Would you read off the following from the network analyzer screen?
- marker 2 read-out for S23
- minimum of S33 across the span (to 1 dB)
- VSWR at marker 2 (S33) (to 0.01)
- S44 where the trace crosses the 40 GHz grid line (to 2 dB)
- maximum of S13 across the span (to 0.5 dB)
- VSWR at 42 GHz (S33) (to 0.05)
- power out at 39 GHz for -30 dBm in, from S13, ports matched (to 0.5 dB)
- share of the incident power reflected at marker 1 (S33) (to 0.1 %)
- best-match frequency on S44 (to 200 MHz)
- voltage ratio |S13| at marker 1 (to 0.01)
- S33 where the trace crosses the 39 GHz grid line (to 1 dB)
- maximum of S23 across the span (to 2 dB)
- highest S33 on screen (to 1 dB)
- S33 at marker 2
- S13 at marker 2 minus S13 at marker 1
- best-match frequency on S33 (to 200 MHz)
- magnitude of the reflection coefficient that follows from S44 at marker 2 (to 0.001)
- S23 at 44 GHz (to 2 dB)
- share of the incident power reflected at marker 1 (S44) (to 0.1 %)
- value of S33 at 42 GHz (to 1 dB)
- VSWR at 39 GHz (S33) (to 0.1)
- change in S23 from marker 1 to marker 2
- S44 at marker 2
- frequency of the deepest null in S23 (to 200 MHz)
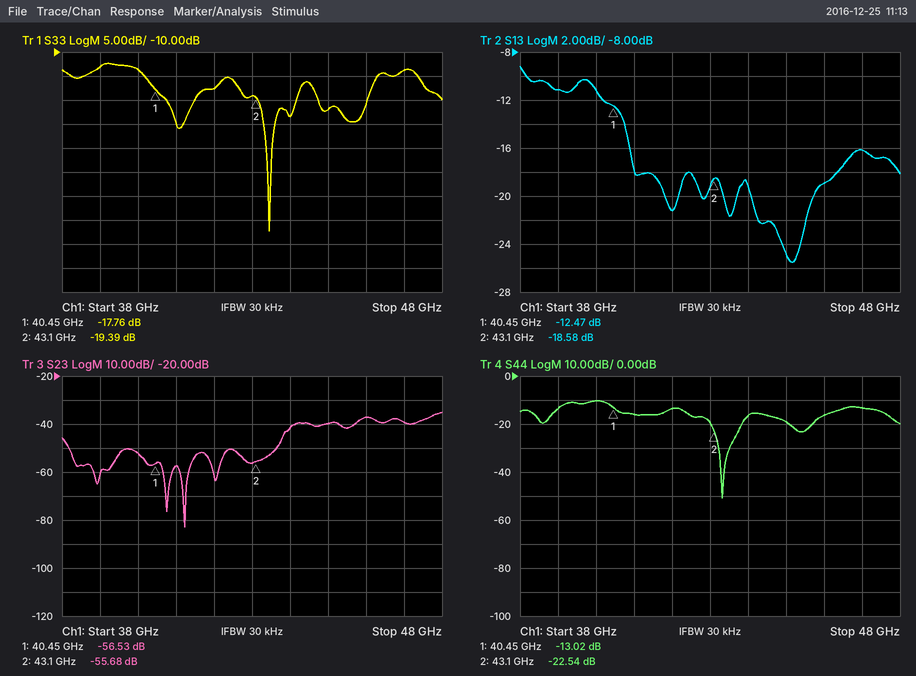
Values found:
-55.68 dB
-47 dB
1.24
-10 dB
-9.0 dB
1.30
-41.0 dBm
1.7 %
43.4 GHz
0.24
-13 dB
-36 dB
-12 dB
-19.39 dB
-6.11 dB
43.4 GHz
0.075
-42 dB
5.0 %
-18 dB
1.6
0.85 dB
-22.54 dB
41.2 GHz
